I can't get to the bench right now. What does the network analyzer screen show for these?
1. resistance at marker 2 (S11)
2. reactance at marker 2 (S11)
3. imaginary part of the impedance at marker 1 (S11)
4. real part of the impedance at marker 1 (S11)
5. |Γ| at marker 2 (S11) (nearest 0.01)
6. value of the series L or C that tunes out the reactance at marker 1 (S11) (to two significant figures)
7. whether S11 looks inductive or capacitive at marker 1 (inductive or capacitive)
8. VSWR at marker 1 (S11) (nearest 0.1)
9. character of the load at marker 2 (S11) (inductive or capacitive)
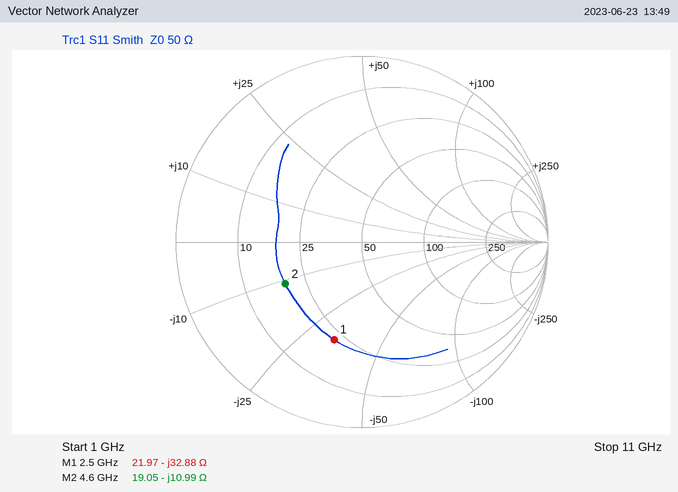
19.05 Ω
-10.99 Ω
-32.88 Ω
21.97 Ω
0.47
2.1 nH
capacitive
3.4
capacitive
